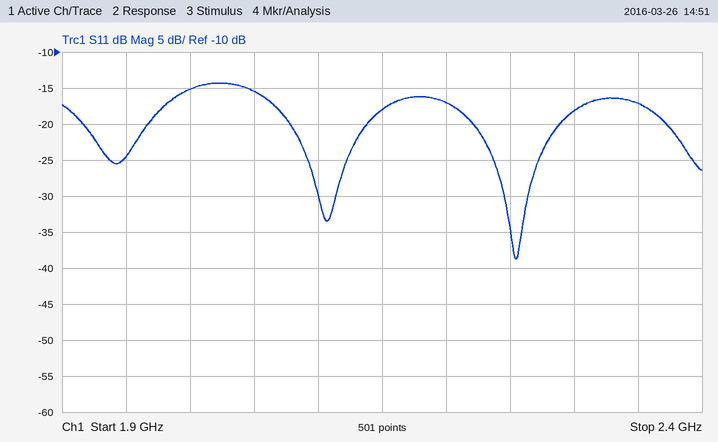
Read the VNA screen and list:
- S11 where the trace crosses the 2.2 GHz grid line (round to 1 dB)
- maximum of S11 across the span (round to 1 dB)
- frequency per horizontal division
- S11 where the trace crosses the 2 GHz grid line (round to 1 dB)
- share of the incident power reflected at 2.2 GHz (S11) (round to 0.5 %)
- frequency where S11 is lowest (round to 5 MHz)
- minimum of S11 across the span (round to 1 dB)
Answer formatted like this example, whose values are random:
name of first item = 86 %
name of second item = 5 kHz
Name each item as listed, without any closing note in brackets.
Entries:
S11 where the trace crosses the 2.2 GHz grid line = -17 dB
maximum of S11 across the span = -14 dB
frequency per horizontal division = 50 MHz
S11 where the trace crosses the 2 GHz grid line = -15 dB
share of the incident power reflected at 2.2 GHz (S11) = 2.0 %
frequency where S11 is lowest = 2.255 GHz
minimum of S11 across the span = -39 dB
